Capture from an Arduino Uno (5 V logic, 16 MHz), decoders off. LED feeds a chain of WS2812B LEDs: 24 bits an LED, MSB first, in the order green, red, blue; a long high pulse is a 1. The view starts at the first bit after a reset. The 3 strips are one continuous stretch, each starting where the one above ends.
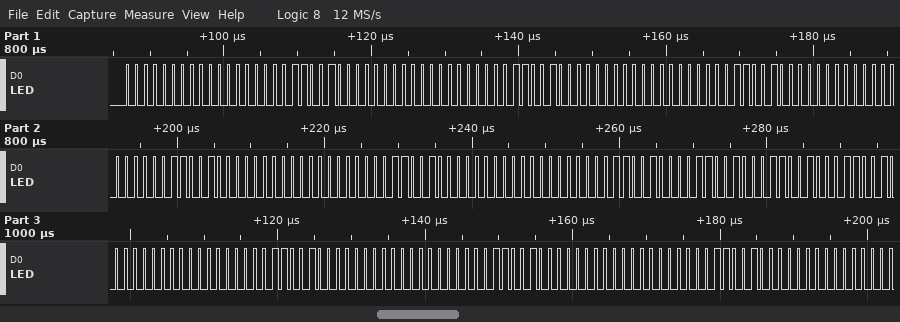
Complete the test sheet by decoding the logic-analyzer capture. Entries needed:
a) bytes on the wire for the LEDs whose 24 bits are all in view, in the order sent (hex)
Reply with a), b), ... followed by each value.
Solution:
a) 00 00 32 00 00 32 00 00 32 00 00 32 00 00 32 00 00 32 19 19 19 00 00 32 00 00 32 00 00 32
